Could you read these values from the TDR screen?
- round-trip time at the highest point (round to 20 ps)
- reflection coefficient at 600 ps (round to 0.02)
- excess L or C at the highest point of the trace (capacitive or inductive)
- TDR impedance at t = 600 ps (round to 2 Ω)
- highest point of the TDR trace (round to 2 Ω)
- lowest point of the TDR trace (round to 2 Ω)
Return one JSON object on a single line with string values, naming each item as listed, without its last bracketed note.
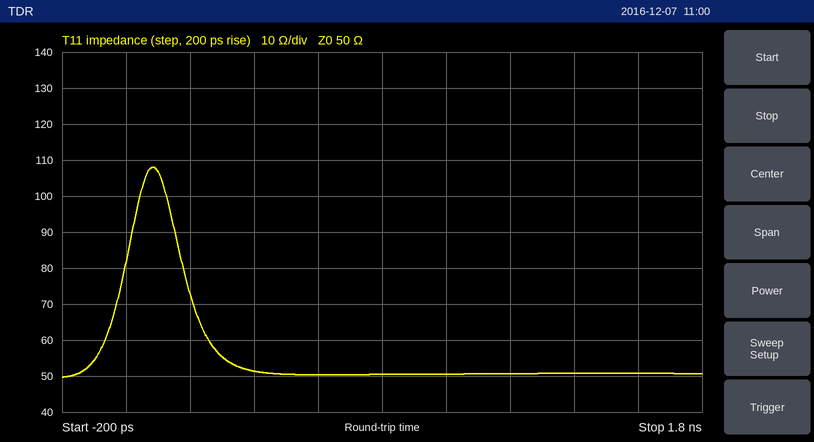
{"round-trip time at the highest point": "80 ps", "reflection coefficient at 600 ps": "0.00", "excess L or C at the highest point of the trace": "inductive", "TDR impedance at t = 600 ps": "50 Ω", "highest point of the TDR trace": "108 Ω", "lowest point of the TDR trace": "50 Ω"}
